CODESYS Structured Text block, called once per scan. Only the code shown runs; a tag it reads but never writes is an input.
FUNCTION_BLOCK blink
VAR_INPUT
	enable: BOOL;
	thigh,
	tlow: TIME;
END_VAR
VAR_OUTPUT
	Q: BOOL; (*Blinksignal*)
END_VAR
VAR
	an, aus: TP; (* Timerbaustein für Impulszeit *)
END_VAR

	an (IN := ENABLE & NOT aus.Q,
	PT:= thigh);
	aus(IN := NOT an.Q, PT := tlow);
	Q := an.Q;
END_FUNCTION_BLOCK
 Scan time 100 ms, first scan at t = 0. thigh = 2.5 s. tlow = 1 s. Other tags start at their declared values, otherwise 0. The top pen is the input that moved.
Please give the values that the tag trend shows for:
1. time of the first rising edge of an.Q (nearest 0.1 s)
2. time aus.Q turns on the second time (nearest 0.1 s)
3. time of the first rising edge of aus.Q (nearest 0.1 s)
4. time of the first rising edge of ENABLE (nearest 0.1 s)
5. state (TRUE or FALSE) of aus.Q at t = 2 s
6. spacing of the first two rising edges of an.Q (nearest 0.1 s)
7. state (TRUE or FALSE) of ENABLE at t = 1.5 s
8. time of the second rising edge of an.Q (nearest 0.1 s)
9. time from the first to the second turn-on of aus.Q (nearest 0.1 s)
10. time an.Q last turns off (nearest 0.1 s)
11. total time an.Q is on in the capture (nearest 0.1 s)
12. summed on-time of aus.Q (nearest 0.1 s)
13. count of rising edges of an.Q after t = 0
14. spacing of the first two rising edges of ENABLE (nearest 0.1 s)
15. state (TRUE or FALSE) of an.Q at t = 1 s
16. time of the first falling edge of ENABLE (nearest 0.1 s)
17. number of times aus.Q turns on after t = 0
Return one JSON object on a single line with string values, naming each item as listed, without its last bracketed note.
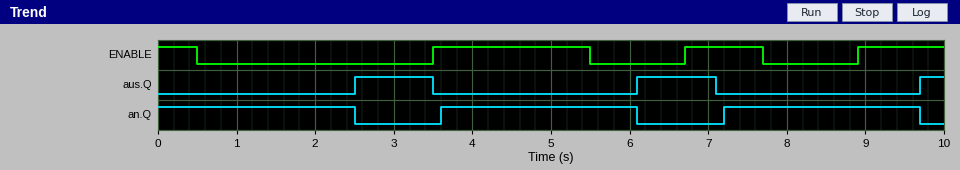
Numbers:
{"time of the first rising edge of an.Q": "3.6 s", "time aus.Q turns on the second time": "6.1 s", "time of the first rising edge of aus.Q": "2.5 s", "time of the first rising edge of ENABLE": "3.5 s", "state (TRUE or FALSE) of aus.Q at t = 2 s": "FALSE", "spacing of the first two rising edges of an.Q": "3.6 s", "state (TRUE or FALSE) of ENABLE at t = 1.5 s": "FALSE", "time of the second rising edge of an.Q": "7.2 s", "time from the first to the second turn-on of aus.Q": "3.6 s", "time an.Q last turns off": "9.7 s", "total time an.Q is on in the capture": "7.5 s", "summed on-time of aus.Q": "2.3 s", "count of rising edges of an.Q after t = 0": "2", "spacing of the first two rising edges of ENABLE": "3.2 s", "state (TRUE or FALSE) of an.Q at t = 1 s": "TRUE", "time of the first falling edge of ENABLE": "0.5 s", "number of times aus.Q turns on after t = 0": "3"}
